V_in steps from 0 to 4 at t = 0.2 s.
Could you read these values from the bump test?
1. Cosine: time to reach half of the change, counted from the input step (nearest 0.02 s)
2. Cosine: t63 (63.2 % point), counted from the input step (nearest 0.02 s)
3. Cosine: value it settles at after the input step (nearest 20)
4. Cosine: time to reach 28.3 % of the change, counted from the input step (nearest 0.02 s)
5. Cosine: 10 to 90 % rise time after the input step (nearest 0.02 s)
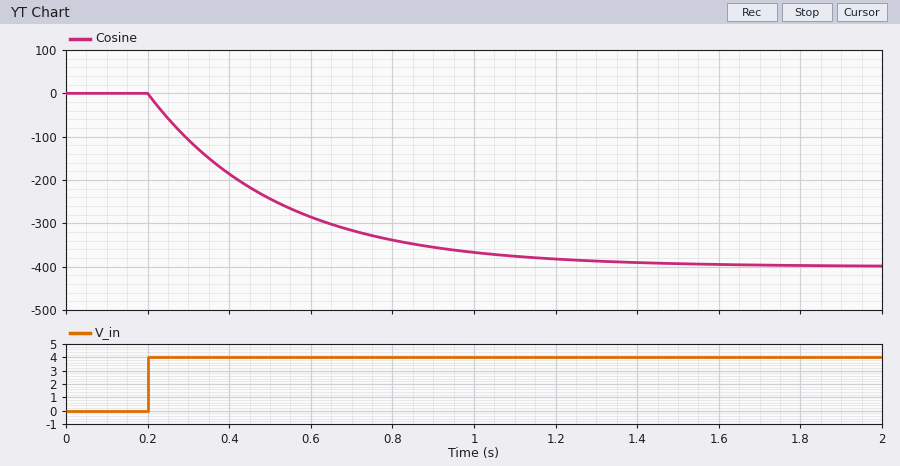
0.22 s
0.32 s
-400
0.10 s
0.70 s
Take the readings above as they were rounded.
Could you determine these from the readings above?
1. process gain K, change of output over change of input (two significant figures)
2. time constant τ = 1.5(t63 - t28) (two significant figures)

-100
0.33 s
